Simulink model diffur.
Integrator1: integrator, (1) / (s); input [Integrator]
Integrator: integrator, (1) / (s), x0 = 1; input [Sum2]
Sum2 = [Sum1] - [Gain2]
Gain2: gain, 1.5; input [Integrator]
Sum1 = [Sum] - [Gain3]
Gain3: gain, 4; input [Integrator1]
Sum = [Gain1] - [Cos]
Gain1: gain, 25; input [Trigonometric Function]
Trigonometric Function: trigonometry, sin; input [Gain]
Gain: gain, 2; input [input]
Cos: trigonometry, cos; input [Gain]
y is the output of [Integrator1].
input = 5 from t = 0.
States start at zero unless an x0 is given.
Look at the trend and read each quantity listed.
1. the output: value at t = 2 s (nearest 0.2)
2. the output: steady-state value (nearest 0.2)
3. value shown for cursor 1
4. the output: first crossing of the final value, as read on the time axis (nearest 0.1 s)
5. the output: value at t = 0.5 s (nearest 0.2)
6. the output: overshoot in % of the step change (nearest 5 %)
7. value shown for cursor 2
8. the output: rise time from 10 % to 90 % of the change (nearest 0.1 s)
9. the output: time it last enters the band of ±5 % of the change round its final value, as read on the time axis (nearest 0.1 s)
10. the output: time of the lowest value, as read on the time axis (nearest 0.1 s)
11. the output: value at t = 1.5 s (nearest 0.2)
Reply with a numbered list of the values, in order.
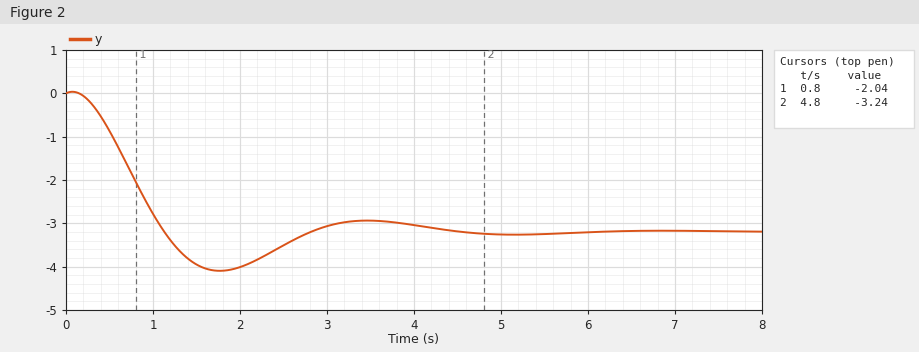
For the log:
1. -4.0
2. -3.2
3. -2.04
4. 1.1 s
5. -0.8
6. 30 %
7. -3.24
8. 0.7 s
9. 4.0 s
10. 1.8 s
11. -4.0
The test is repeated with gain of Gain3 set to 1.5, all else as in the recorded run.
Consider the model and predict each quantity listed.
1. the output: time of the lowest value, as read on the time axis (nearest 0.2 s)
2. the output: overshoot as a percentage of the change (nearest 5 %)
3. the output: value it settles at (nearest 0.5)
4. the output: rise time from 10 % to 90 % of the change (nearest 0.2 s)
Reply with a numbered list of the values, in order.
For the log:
1. 3.4 s
2. 10 %
3. -8.5
4. 1.6 s
